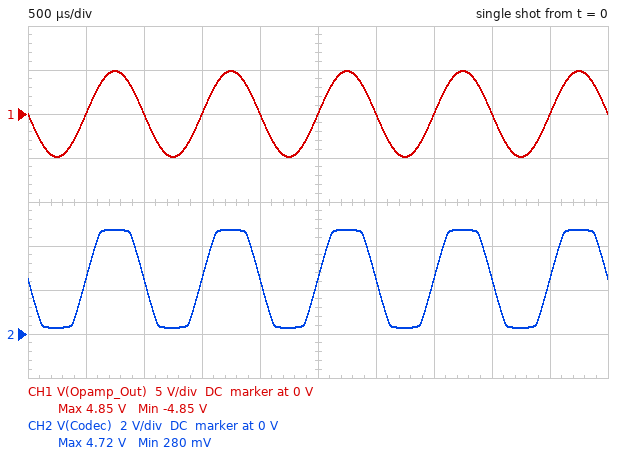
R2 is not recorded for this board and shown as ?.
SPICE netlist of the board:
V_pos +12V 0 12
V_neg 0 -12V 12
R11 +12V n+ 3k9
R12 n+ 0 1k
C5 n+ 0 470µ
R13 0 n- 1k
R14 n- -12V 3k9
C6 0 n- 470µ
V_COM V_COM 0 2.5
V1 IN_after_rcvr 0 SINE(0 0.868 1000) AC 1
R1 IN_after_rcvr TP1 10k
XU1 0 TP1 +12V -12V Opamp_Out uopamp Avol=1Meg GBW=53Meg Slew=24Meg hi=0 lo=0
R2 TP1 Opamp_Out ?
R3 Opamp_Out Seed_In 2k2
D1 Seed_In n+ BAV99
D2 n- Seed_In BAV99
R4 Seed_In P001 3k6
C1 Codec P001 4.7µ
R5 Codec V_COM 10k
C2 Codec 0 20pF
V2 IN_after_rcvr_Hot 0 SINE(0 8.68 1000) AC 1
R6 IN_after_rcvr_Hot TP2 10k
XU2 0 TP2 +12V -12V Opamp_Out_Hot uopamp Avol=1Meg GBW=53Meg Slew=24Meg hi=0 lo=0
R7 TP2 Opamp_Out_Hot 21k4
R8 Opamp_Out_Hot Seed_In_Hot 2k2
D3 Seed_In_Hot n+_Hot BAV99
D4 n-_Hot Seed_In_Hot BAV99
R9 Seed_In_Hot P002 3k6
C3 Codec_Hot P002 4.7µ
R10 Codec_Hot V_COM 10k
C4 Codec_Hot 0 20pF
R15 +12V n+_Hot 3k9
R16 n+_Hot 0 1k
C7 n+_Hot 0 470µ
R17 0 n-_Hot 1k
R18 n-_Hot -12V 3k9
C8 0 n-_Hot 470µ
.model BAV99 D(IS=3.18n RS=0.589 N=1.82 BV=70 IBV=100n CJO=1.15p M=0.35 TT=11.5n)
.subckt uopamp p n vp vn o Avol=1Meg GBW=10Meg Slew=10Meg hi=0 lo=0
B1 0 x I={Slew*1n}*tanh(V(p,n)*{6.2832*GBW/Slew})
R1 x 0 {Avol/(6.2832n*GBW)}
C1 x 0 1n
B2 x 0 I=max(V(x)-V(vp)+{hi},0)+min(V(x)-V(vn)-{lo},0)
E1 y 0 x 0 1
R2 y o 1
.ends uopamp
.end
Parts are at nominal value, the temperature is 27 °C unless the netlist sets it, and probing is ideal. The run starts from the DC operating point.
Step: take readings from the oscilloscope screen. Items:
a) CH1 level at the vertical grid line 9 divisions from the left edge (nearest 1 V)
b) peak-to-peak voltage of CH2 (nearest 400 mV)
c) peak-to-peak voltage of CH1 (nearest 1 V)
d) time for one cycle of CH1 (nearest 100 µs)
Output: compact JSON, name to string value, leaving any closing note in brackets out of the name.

{"CH1 level at the vertical grid line 9 divisions from the left edge": "0 V", "peak-to-peak voltage of CH2": "4.4 V", "peak-to-peak voltage of CH1": "10 V", "time for one cycle of CH1": "1.0 ms"}
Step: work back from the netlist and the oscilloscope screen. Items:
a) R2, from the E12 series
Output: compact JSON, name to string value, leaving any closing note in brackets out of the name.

{"R2, from the E12 series": "56 kΩ"}
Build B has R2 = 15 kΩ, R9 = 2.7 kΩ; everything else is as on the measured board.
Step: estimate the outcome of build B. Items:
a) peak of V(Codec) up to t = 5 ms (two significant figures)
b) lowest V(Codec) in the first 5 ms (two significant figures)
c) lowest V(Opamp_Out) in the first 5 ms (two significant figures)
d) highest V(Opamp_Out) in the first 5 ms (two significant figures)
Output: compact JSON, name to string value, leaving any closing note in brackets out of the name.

{"peak of V(Codec) up to t = 5 ms": "3.3 V", "lowest V(Codec) in the first 5 ms": "1.7 V", "lowest V(Opamp_Out) in the first 5 ms": "-1.3 V", "highest V(Opamp_Out) in the first 5 ms": "1.3 V"}
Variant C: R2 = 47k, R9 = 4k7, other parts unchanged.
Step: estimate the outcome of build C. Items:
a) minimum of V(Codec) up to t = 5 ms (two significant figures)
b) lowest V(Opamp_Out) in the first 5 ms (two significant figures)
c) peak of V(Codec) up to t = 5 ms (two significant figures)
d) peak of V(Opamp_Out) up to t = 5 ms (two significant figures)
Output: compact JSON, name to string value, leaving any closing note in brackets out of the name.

{"minimum of V(Codec) up to t = 5 ms": "310 mV", "lowest V(Opamp_Out) in the first 5 ms": "-4.1 V", "peak of V(Codec) up to t = 5 ms": "4.7 V", "peak of V(Opamp_Out) up to t = 5 ms": "4.1 V"}
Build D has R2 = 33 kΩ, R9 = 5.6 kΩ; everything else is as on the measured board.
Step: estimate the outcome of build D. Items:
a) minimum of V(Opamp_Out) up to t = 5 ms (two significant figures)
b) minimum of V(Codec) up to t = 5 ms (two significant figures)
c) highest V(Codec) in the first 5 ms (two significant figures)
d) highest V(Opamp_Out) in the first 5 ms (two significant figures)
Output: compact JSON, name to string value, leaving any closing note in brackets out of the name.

{"minimum of V(Opamp_Out) up to t = 5 ms": "-2.9 V", "minimum of V(Codec) up to t = 5 ms": "690 mV", "highest V(Codec) in the first 5 ms": "4.3 V", "highest V(Opamp_Out) in the first 5 ms": "2.9 V"}
